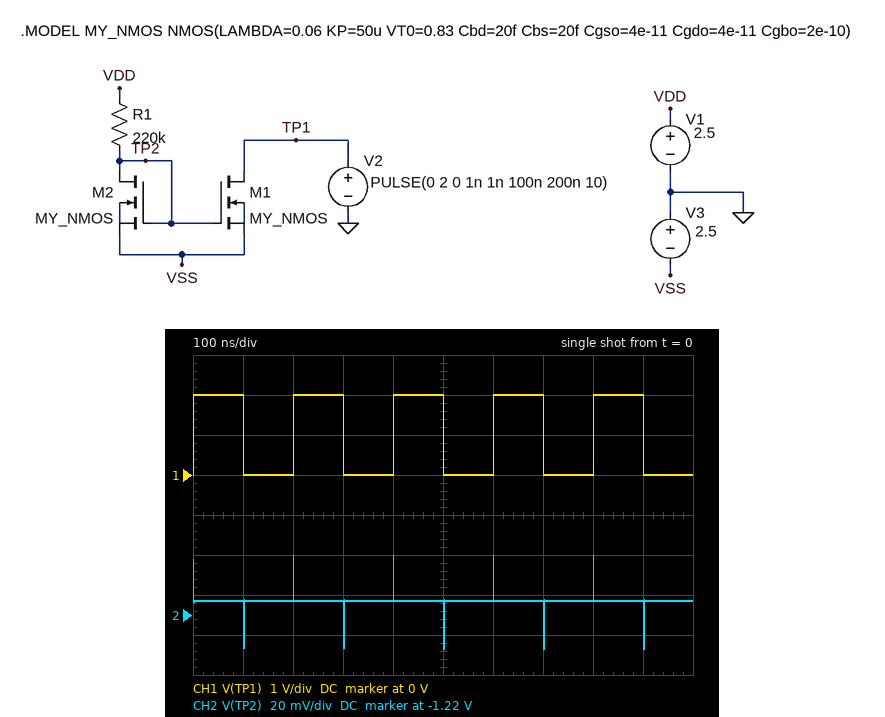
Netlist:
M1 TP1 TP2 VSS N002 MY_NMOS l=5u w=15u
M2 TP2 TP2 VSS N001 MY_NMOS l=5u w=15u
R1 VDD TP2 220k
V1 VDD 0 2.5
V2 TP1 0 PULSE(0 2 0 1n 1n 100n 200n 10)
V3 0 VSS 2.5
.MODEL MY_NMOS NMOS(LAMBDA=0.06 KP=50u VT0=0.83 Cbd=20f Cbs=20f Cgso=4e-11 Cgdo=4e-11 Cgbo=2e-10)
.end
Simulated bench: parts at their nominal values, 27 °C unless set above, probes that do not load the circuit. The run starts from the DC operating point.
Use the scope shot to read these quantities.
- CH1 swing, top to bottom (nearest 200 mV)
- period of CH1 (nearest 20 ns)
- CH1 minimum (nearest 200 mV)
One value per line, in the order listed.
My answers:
2.0 V
200 ns
0 V
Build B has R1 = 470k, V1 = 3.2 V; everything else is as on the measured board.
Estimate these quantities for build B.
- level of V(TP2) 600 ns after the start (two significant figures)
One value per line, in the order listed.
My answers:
-1.3 V
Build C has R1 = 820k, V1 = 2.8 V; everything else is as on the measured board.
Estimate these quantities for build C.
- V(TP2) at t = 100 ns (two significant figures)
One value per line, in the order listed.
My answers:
-1.4 V
